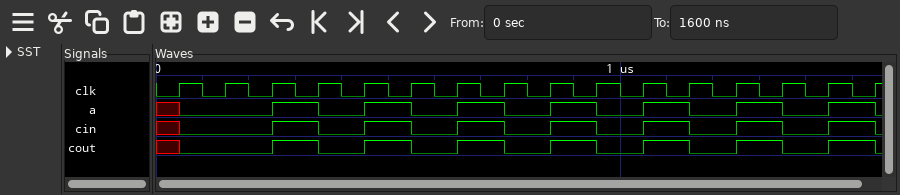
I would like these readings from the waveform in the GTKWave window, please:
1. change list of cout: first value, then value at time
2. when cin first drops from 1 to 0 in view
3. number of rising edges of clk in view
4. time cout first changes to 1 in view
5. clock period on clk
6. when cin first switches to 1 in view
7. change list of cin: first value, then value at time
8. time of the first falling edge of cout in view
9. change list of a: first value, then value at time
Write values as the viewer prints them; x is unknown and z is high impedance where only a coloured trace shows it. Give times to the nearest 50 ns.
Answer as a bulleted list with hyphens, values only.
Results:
- x, 0 at 50 ns, 1 at 250 ns, 0 at 350 ns, 1 at 450 ns, 0 at 550 ns, 1 at 650 ns, 0 at 750 ns, 1 at 850 ns, 0 at 950 ns, 1 at 1050 ns, 0 at 1150 ns, 1 at 1250 ns, 0 at 1350 ns, 1 at 1450 ns, 0 at 1550 ns
- 350 ns
- 16
- 250 ns
- 100 ns
- 250 ns
- x, 0 at 50 ns, 1 at 250 ns, 0 at 350 ns, 1 at 450 ns, 0 at 550 ns, 1 at 650 ns, 0 at 750 ns, 1 at 850 ns, 0 at 950 ns, 1 at 1050 ns, 0 at 1150 ns, 1 at 1250 ns, 0 at 1350 ns, 1 at 1450 ns, 0 at 1550 ns
- 350 ns
- x, 0 at 50 ns, 1 at 250 ns, 0 at 350 ns, 1 at 450 ns, 0 at 550 ns, 1 at 650 ns, 0 at 750 ns, 1 at 850 ns, 0 at 950 ns, 1 at 1050 ns, 0 at 1150 ns, 1 at 1250 ns, 0 at 1350 ns, 1 at 1450 ns, 0 at 1550 ns
